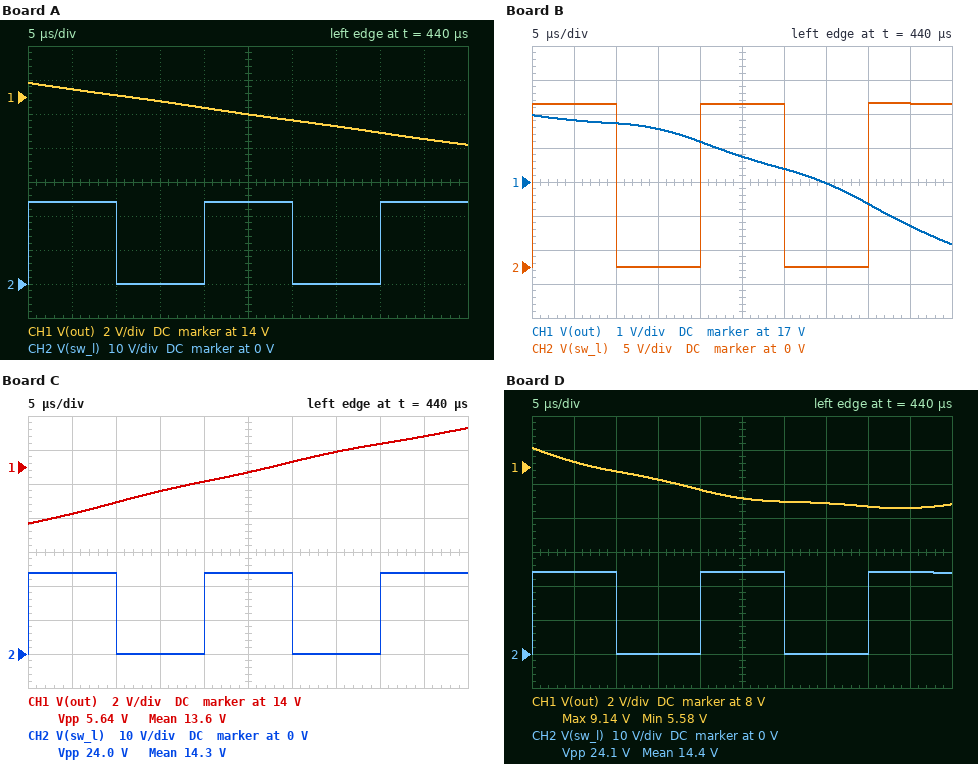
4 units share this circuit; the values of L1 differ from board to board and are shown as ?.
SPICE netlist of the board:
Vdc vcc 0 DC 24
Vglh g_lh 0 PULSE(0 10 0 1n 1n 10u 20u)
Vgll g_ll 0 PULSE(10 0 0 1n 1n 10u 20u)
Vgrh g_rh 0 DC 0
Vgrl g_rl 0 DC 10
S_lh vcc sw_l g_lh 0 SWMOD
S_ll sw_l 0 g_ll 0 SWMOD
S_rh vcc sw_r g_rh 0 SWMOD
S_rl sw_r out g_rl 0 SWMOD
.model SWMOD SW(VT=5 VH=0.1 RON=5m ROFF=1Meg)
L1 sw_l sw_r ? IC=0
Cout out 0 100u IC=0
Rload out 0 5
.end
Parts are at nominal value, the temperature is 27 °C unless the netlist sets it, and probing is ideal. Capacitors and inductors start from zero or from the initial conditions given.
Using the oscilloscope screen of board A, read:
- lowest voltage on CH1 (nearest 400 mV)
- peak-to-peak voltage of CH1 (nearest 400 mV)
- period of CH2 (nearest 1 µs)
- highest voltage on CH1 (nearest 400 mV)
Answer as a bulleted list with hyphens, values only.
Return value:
- 11.2 V
- 3.6 V
- 20 µs
- 14.8 V
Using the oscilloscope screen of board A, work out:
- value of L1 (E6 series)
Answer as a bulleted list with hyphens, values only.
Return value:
- 100 µH
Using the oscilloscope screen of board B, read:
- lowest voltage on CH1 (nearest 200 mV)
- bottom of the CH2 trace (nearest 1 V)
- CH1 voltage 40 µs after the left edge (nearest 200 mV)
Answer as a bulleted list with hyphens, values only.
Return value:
- 15.2 V
- 0 V
- 16.4 V
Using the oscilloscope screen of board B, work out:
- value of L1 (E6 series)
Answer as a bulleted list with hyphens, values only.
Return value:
- 22 µH
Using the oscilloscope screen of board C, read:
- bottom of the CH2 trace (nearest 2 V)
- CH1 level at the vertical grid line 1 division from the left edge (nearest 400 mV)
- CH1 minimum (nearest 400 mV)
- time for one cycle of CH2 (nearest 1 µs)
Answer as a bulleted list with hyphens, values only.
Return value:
- 0 V
- 11.2 V
- 10.8 V
- 20 µs
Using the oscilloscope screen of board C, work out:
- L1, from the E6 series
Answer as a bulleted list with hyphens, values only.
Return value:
- 33 µH
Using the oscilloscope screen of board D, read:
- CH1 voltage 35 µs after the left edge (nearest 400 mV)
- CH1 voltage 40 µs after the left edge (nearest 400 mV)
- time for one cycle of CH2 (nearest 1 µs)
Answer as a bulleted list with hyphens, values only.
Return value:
- 6.0 V
- 5.6 V
- 20 µs
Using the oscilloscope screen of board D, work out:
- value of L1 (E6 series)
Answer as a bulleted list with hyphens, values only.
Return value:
- 15 µH
